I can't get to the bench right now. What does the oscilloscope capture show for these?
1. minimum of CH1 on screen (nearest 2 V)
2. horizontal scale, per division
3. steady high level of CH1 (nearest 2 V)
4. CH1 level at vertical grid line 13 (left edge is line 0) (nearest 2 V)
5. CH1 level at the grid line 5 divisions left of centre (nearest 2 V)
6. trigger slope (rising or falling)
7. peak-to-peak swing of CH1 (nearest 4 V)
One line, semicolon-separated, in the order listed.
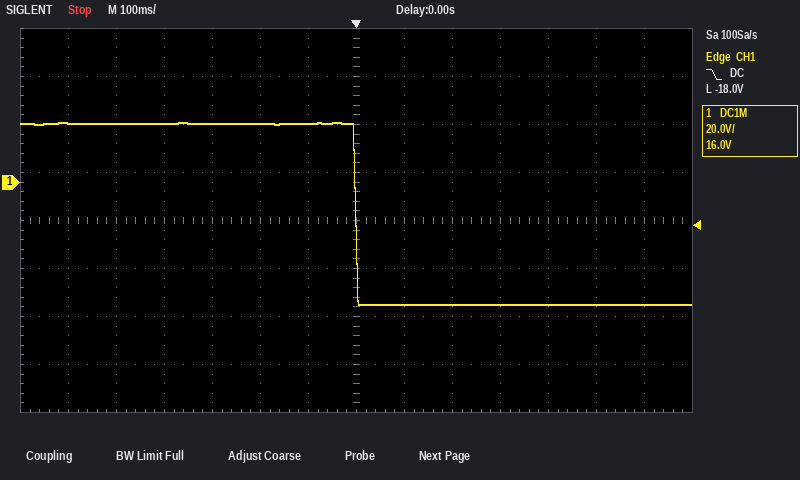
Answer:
-52 V; 100 ms; 24 V; -52 V; 24 V; falling; 76 V
